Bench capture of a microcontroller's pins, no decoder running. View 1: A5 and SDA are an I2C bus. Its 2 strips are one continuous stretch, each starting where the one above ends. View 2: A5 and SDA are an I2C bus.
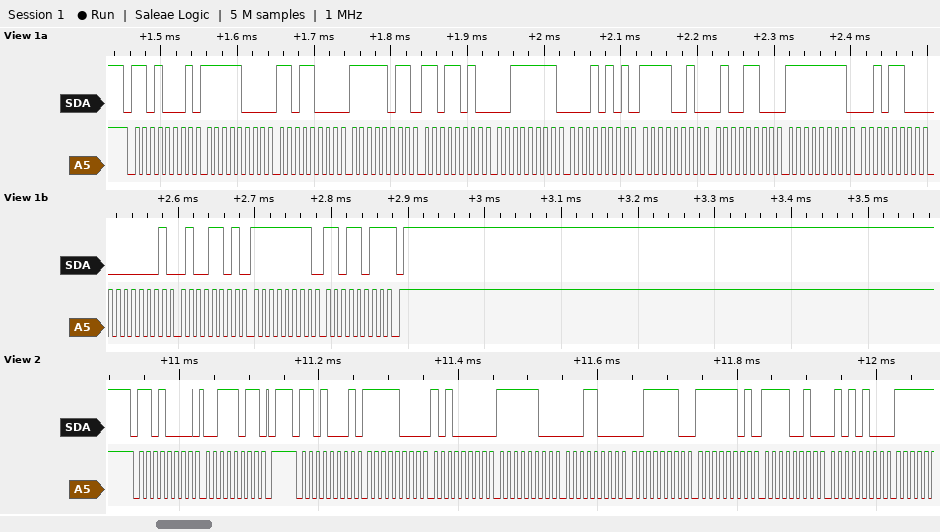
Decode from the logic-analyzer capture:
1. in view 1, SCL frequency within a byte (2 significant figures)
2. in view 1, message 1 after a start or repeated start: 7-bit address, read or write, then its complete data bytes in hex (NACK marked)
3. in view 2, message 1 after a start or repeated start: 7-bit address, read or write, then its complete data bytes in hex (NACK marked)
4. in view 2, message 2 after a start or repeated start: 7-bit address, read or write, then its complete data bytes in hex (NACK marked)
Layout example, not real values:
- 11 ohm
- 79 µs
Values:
- 100 kHz
- 0x68 read: F8 D8 FB DA 3F 15 F2 4C FF 2C 01 4D FF DB NACK
- 0x68 write: 3B
- 0x68 read: F8 A0 FC 18 3E FD F2 54
